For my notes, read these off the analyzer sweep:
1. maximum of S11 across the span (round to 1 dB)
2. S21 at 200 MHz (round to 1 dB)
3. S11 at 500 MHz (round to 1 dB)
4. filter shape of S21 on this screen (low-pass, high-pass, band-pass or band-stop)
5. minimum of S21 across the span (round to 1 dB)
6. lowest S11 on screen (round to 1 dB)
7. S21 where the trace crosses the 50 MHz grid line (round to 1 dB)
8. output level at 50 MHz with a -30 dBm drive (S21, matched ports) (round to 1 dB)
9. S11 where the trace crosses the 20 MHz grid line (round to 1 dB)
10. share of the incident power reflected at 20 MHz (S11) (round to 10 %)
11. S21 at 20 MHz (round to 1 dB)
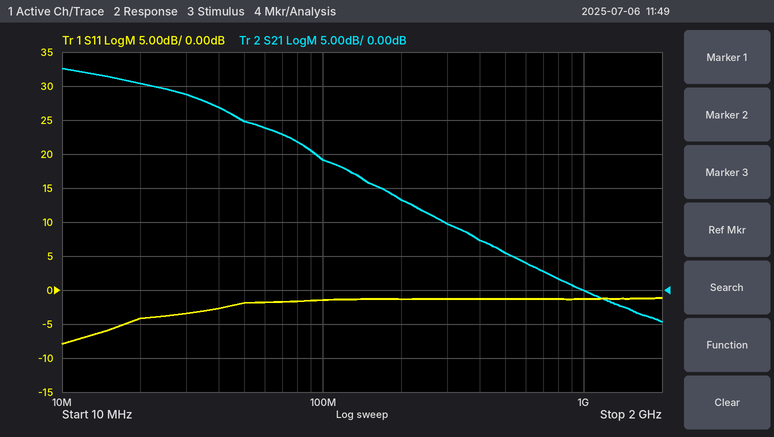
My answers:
-1 dB
13 dB
-1 dB
low-pass
-5 dB
-8 dB
25 dB
-5 dBm
-4 dB
40 %
30 dB
